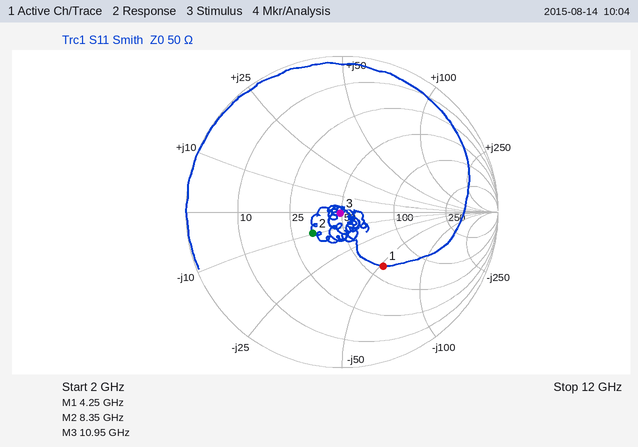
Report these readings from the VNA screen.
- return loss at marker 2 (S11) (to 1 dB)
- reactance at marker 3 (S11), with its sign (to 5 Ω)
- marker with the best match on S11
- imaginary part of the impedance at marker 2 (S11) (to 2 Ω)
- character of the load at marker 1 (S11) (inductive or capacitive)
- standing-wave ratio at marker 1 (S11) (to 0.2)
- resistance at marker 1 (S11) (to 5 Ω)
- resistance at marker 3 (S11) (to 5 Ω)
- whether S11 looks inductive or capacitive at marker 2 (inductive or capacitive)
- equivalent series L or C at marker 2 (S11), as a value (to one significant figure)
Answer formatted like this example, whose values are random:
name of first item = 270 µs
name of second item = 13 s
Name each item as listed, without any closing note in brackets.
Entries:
return loss at marker 2 (S11) = 13 dB
reactance at marker 3 (S11), with its sign = 0 Ω
marker with the best match on S11 = marker 3
imaginary part of the impedance at marker 2 (S11) = -10 Ω
character of the load at marker 1 (S11) = capacitive
standing-wave ratio at marker 1 (S11) = 2.6
resistance at marker 1 (S11) = 60 Ω
resistance at marker 3 (S11) = 50 Ω
whether S11 looks inductive or capacitive at marker 2 = capacitive
equivalent series L or C at marker 2 (S11), as a value = 2 pF
